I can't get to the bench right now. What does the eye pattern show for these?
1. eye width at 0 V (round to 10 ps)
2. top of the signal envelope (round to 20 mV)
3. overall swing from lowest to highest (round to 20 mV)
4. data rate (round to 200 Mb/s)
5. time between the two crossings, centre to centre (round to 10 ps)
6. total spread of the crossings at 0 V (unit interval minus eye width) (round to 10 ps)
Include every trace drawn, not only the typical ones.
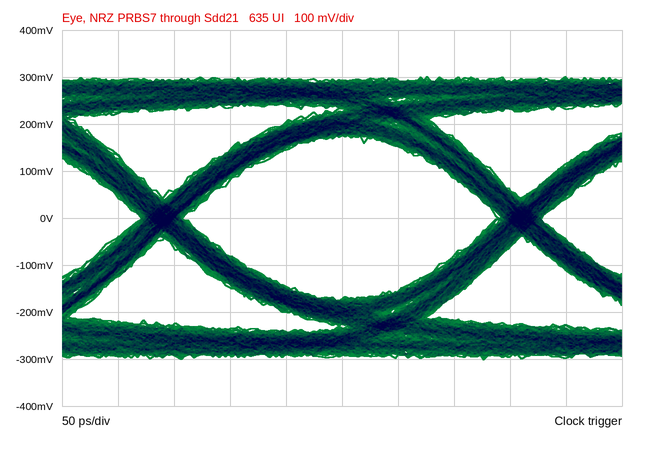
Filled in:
280 ps
300 mV
600 mV
3.2 Gb/s
320 ps
40 ps
